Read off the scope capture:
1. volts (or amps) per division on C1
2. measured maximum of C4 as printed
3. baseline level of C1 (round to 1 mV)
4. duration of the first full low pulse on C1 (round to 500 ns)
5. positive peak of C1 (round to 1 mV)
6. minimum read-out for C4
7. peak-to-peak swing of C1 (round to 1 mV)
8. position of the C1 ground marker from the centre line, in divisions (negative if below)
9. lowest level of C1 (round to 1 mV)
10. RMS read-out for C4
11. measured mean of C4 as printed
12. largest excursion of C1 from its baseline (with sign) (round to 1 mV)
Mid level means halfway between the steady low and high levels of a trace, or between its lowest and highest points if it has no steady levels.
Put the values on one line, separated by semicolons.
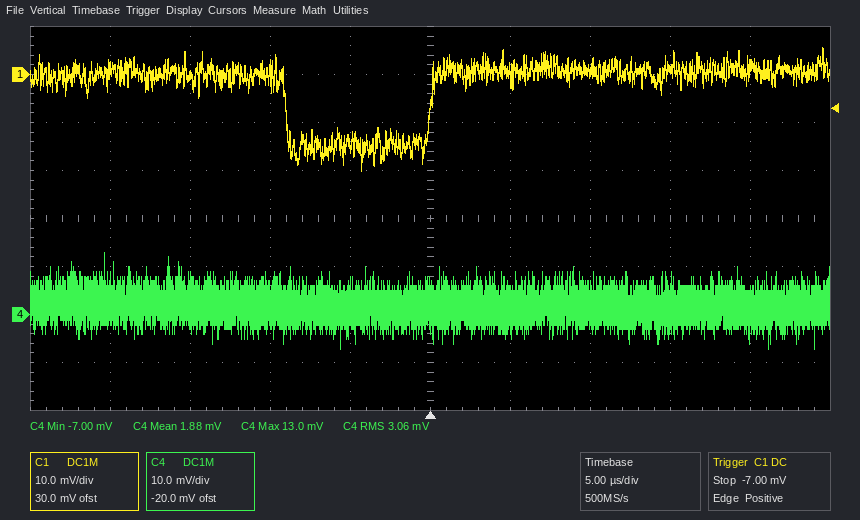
10 mV; 13.0 mV; 0 mV; 9.0 µs; 6 mV; -7.00 mV; 26 mV; +3.0 div; -20 mV; 3.06 mV; 1.88 mV; -20 mV
